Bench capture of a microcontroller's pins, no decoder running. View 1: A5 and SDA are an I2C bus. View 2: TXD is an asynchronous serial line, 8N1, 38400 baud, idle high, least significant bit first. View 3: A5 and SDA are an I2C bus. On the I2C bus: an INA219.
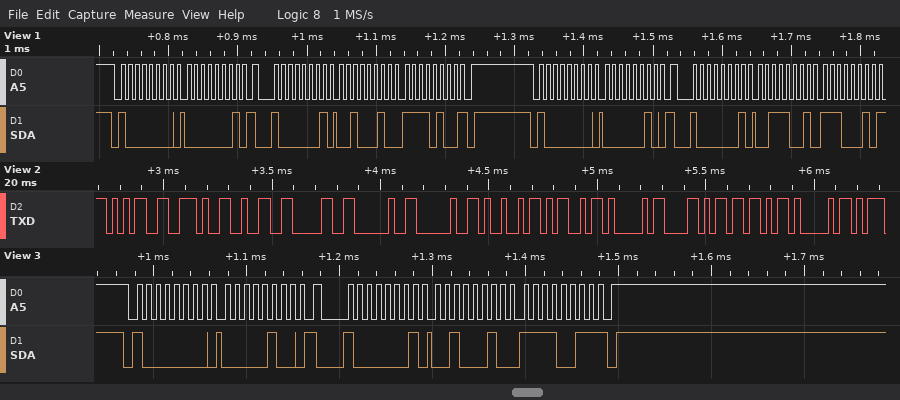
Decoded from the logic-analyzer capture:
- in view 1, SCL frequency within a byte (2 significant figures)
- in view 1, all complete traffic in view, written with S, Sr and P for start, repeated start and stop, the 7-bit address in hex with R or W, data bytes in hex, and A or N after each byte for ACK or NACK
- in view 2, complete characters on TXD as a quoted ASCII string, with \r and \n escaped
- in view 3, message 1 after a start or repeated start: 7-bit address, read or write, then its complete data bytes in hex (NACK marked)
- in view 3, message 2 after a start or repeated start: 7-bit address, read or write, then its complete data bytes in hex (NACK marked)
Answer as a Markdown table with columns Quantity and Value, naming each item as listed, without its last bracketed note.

| Quantity | Value |
|---|---|
| in view 1, SCL frequency within a byte | 100 kHz |
| in view 1, all complete traffic in view, written with S, Sr and P for start, repeated start and stop, the 7-bit address in hex with R or W, data bytes in hex, and A or N after each byte for ACK or NACK | S 40W A 01 A Sr 40R A 22 A F4 N P S 40W A 02 A Sr 40R A 39 A E2 N |
| in view 2, complete characters on TXD as a quoted ASCII string, with \r and \n escaped | "5.20  IMAX[A" |
| in view 3, message 1 after a start or repeated start: 7-bit address, read or write, then its complete data bytes in hex | 0x40 write: 04 |
| in view 3, message 2 after a start or repeated start: 7-bit address, read or write, then its complete data bytes in hex | 0x40 read: 22 F3 NACK |
